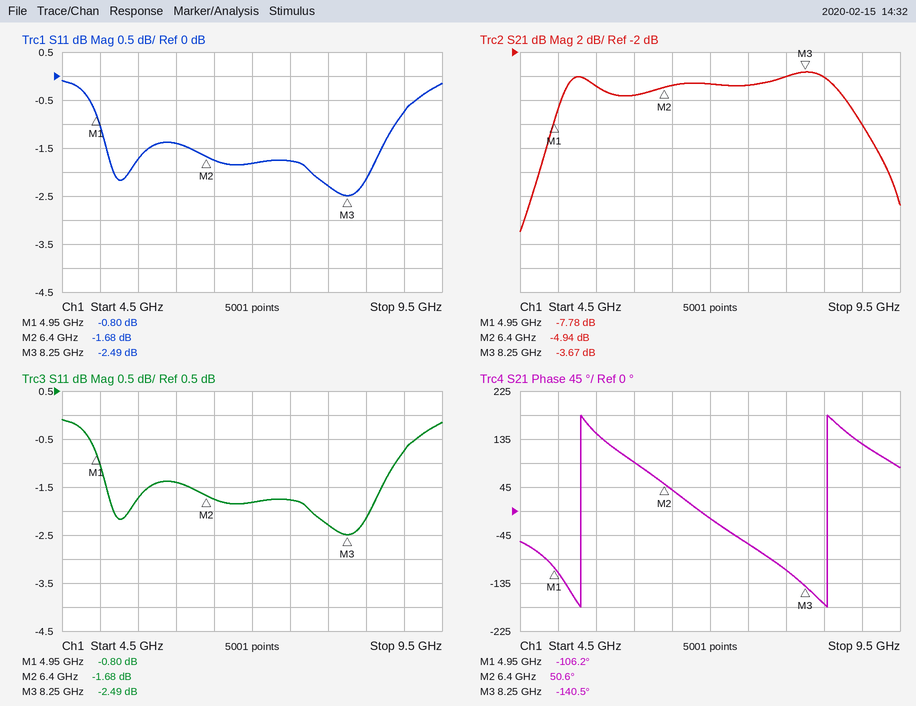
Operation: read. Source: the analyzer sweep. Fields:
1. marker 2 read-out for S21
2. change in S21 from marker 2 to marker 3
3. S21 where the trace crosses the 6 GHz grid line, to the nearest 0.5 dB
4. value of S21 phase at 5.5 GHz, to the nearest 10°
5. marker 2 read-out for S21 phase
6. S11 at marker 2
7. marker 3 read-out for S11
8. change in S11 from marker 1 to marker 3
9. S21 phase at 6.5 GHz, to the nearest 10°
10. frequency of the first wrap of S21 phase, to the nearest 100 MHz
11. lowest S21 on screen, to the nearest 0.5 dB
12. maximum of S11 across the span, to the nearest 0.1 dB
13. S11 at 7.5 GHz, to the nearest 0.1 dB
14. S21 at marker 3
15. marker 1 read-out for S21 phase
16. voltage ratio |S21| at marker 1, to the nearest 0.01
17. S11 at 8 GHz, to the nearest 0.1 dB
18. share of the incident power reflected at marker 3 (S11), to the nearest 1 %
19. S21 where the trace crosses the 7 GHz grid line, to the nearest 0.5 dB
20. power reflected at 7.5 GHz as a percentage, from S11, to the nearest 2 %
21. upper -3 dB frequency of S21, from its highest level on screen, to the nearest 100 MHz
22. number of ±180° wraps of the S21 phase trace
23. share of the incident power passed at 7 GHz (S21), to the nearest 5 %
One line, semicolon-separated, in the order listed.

-4.94 dB; 1.27 dB; -5.5 dB; 150°; 50.6°; -1.68 dB; -2.49 dB; -1.69 dB; 40°; 5.3 GHz; -17.0 dB; -0.1 dB; -1.8 dB; -3.67 dB; -106.2°; 0.41; -2.3 dB; 56 %; -4.5 dB; 66 %; 8.9 GHz; 2; 35 %
